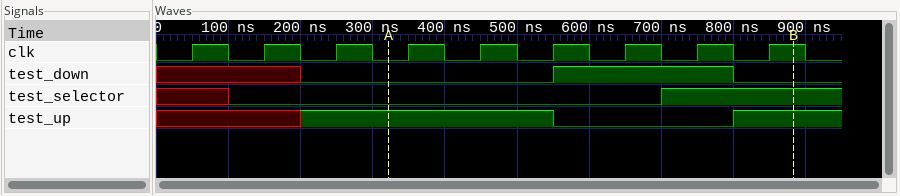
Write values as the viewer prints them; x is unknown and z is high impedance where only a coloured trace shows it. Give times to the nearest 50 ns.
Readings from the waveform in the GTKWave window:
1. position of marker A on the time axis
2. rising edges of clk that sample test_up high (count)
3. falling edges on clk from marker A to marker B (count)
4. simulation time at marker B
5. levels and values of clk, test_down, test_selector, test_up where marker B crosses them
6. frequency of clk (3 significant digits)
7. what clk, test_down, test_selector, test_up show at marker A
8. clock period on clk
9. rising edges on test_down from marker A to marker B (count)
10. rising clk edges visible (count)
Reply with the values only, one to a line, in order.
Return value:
300 ns
5
5
900 ns
clk=1, test_down=0, test_selector=1, test_up=1
10.0 MHz
clk=0, test_down=0, test_selector=0, test_up=1
100 ns
1
9
